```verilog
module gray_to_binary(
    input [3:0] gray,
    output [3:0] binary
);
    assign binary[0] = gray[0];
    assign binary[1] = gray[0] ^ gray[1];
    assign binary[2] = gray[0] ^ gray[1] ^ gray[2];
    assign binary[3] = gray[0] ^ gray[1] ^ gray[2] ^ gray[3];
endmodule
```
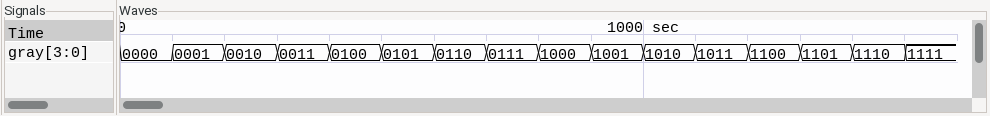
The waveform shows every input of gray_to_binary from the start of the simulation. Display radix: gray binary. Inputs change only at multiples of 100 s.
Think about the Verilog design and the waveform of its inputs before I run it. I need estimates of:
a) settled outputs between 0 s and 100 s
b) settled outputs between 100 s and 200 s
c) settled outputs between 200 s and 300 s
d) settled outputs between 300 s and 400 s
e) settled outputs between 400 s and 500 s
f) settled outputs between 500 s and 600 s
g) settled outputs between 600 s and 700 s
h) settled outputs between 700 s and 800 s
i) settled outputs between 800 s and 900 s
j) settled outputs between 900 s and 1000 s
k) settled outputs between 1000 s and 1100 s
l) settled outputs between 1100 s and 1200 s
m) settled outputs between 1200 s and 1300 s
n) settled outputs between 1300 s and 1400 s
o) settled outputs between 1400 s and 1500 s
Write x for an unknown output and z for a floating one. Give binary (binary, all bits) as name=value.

binary=0000
binary=1111
binary=1110
binary=0001
binary=1100
binary=0011
binary=0010
binary=1101
binary=1000
binary=0111
binary=0110
binary=1001
binary=0100
binary=1011
binary=1010
